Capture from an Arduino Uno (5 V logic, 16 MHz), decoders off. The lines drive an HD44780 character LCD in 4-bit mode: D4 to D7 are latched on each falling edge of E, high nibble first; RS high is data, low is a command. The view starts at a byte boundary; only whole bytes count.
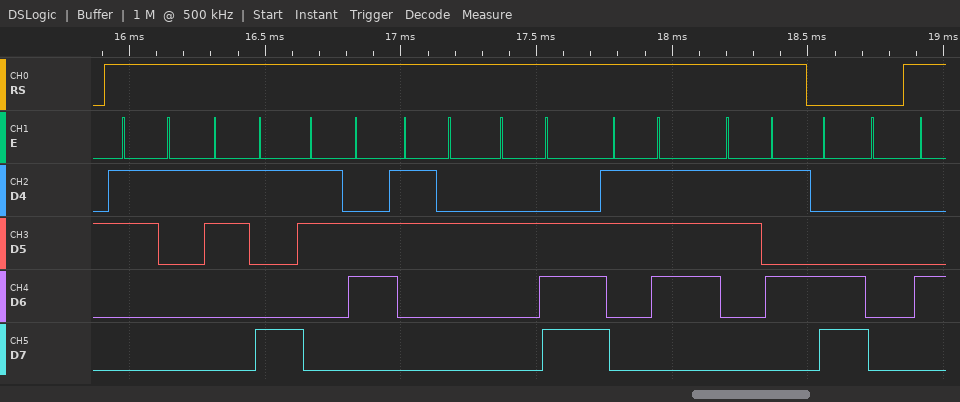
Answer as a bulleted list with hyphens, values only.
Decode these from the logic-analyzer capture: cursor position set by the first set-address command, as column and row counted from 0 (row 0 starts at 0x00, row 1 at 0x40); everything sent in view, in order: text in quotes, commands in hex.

- column 0, row 1
- "1962.75" 0xC0
